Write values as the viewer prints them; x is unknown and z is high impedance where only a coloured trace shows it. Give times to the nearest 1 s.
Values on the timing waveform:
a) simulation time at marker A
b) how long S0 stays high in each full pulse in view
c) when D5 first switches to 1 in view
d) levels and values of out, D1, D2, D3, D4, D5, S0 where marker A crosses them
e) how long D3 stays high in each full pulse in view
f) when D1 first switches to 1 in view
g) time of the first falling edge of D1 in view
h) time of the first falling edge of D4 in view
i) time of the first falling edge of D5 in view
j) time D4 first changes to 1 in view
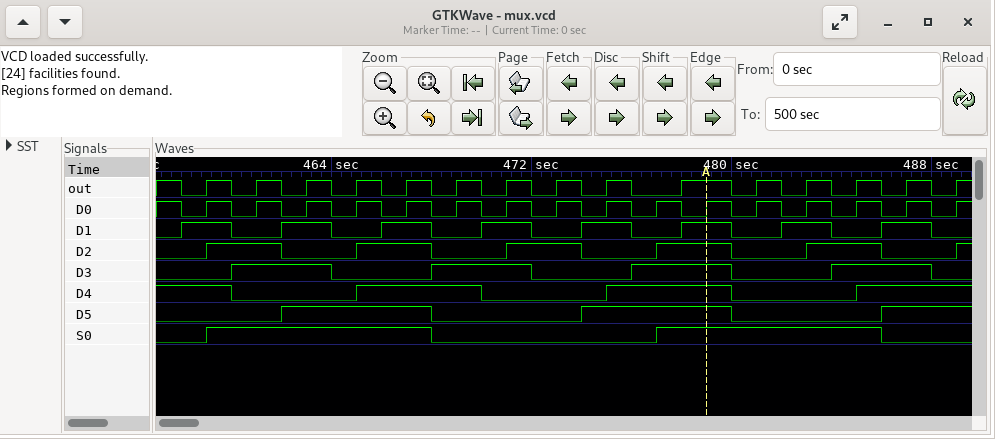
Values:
479 s
9 s, 9 s
462 s
out=1, D1=1, D2=1, D3=1, D4=1, D5=1, S0=1
4 s, 4 s, 4 s, 4 s
458 s
460 s
460 s
468 s
465 s
